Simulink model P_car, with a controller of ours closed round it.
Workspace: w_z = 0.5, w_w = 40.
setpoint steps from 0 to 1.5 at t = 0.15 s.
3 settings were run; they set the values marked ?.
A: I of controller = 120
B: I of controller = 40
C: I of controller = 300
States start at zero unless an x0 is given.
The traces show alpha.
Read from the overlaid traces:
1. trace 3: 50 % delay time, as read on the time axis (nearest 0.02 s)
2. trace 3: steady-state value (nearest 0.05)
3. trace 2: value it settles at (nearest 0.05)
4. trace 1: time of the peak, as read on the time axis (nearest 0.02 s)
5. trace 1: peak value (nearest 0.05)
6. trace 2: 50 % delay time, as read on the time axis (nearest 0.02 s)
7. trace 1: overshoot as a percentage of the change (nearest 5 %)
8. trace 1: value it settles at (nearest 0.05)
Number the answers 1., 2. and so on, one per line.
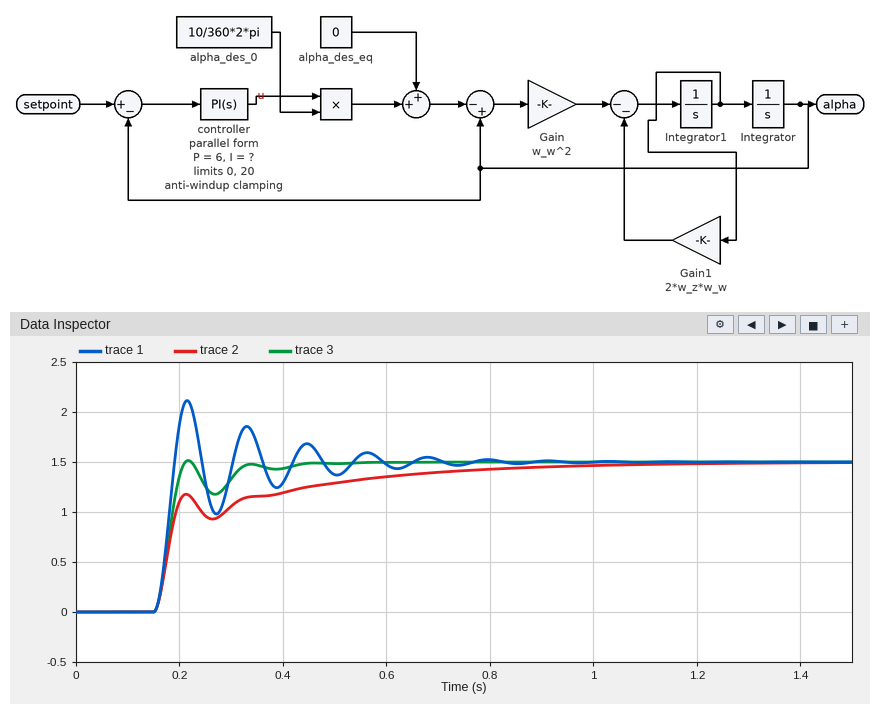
1. 0.18 s
2. 1.50
3. 1.50
4. 0.22 s
5. 2.10
6. 0.18 s
7. 40 %
8. 1.50
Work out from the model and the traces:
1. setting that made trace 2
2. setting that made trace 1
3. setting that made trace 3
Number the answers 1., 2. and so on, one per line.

1. B
2. C
3. A
